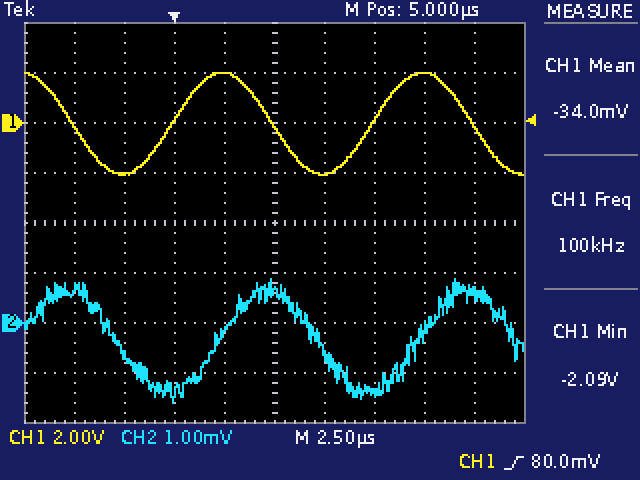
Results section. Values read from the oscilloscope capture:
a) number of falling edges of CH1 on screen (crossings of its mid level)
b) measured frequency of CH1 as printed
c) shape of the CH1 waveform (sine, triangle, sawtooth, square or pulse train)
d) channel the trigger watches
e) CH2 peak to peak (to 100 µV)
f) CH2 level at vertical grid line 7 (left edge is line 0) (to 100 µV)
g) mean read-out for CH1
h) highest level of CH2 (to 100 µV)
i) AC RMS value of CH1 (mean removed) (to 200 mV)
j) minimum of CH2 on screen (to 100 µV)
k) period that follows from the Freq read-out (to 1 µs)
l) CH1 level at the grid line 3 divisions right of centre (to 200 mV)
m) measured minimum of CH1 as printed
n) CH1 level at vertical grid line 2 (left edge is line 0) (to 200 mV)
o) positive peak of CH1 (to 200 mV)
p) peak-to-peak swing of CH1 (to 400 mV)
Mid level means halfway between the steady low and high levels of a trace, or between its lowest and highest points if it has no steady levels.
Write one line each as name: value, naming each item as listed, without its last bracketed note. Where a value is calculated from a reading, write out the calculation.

number of falling edges of CH1 on screen: 3
measured frequency of CH1 as printed: 100 kHz
shape of the CH1 waveform: sine
channel the trigger watches: CH1
CH2 peak to peak: 900 µV − (-1.6 mV) = 2.5 mV
CH2 level at vertical grid line 7 (left edge is line 0): -1.4 mV
mean read-out for CH1: -34.0 mV
highest level of CH2: 900 µV
AC RMS value of CH1 (mean removed): 4.0 V / (2√2) ≈ 1.4 V
minimum of CH2 on screen: -1.6 mV
period that follows from the Freq read-out: 1 / 100 kHz ≈ 10 µs
CH1 level at the grid line 3 divisions right of centre: 2.0 V
measured minimum of CH1 as printed: -2.09 V
CH1 level at vertical grid line 2 (left edge is line 0): -2.0 V
positive peak of CH1: 2.0 V
peak-to-peak swing of CH1: 4.0 V
